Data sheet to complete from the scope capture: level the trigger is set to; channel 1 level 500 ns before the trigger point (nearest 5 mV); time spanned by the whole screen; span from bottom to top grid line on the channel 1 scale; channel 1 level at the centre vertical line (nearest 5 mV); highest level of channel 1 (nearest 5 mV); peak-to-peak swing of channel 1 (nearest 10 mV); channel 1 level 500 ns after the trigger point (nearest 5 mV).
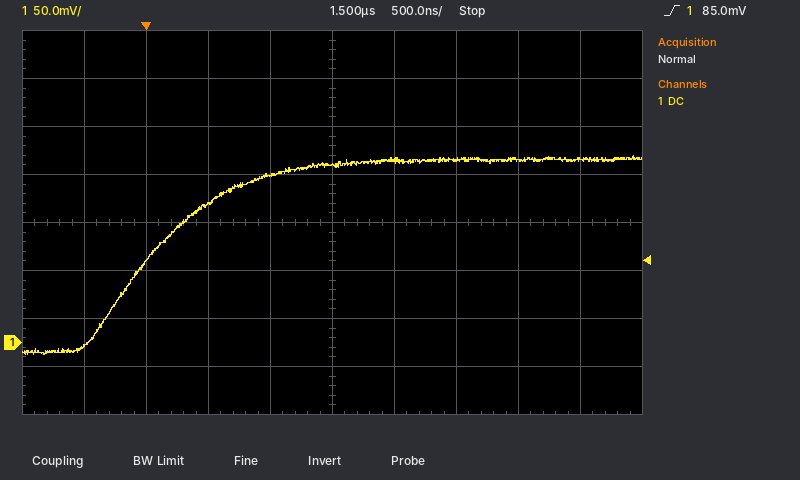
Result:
85.0 mV
-5 mV
5 µs
400 mV
185 mV
195 mV
210 mV
145 mV
